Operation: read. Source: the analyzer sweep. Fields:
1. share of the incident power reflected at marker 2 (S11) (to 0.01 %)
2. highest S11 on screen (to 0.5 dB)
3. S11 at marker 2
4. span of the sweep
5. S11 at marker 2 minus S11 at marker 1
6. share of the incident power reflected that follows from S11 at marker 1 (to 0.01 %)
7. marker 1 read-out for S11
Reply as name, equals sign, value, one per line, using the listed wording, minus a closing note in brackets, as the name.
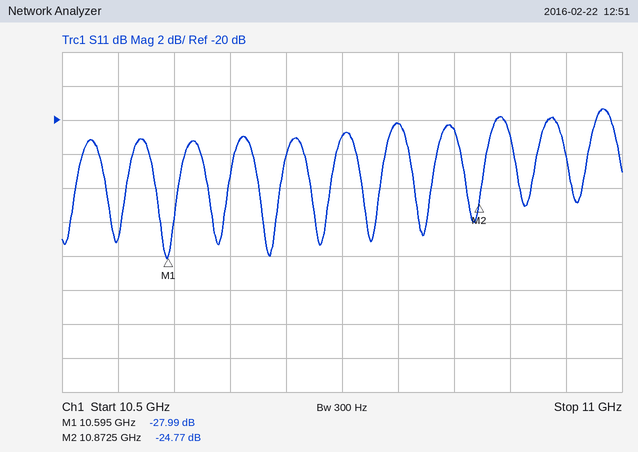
share of the incident power reflected at marker 2 (S11) = 0.33 %
highest S11 on screen = -19.5 dB
S11 at marker 2 = -24.77 dB
span of the sweep = 500 MHz
S11 at marker 2 minus S11 at marker 1 = 3.22 dB
share of the incident power reflected that follows from S11 at marker 1 = 0.16 %
marker 1 read-out for S11 = -27.99 dB
